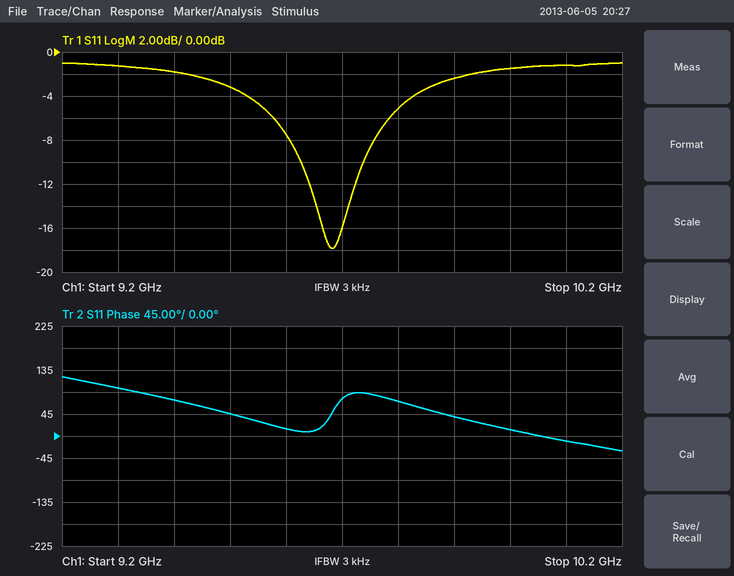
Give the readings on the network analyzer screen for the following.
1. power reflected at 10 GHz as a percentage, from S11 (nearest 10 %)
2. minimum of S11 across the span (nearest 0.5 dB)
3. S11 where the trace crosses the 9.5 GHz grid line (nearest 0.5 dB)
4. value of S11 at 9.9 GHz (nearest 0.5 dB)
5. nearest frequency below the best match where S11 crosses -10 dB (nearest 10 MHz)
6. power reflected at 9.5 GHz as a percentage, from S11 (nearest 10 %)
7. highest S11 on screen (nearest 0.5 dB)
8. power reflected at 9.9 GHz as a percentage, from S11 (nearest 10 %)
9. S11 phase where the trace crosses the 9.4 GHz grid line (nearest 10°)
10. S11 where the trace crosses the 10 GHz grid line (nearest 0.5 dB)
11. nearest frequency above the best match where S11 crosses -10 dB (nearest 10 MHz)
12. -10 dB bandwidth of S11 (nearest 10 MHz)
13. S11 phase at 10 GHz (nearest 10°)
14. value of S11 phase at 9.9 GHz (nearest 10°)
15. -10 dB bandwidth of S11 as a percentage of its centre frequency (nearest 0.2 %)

70 %
-18.0 dB
-3.0 dB
-2.5 dB
9.63 GHz
50 %
-1.0 dB
60 %
70°
-1.5 dB
9.74 GHz
110 MHz
10°
40°
1.2 %
